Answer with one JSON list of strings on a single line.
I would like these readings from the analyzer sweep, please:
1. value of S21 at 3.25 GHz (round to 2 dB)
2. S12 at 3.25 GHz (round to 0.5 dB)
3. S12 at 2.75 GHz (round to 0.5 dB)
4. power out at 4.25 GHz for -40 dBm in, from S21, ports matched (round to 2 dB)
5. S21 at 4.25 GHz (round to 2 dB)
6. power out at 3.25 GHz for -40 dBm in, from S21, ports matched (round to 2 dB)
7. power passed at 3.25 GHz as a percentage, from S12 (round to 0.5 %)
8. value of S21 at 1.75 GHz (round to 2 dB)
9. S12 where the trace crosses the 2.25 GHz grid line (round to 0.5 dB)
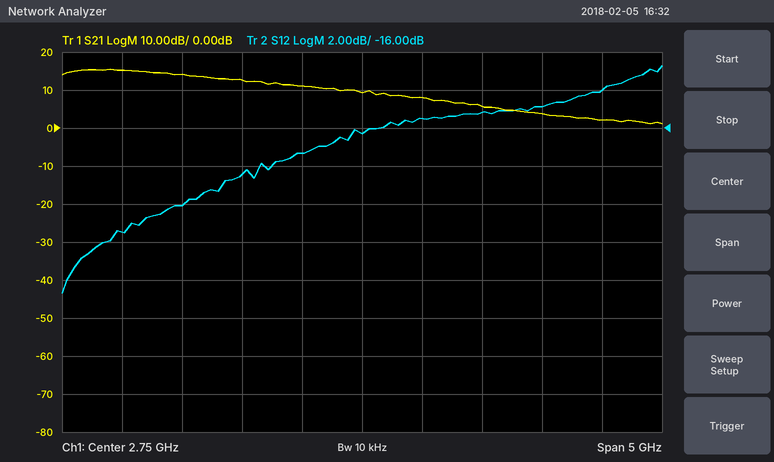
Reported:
["8 dB", "-15.5 dB", "-16.5 dB", "-36 dBm", "4 dB", "-32 dBm", "3.0 %", "12 dB", "-17.5 dB"]
